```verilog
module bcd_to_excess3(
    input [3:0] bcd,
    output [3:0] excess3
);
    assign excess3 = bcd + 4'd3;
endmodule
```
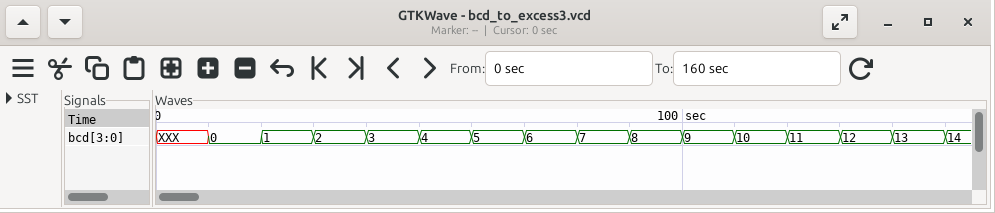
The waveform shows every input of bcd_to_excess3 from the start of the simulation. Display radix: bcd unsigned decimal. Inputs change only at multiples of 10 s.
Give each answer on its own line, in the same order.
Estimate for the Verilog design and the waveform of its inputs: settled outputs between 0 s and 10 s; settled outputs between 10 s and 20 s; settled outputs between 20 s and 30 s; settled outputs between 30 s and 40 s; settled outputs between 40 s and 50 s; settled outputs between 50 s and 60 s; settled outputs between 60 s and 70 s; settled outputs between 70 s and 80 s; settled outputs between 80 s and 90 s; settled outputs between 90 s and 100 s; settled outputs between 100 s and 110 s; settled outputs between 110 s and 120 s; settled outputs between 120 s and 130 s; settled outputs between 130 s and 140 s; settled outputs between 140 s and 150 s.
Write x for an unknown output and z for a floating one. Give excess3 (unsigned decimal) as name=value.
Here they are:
excess3=x
excess3=3
excess3=4
excess3=5
excess3=6
excess3=7
excess3=8
excess3=9
excess3=10
excess3=11
excess3=12
excess3=13
excess3=14
excess3=15
excess3=0
